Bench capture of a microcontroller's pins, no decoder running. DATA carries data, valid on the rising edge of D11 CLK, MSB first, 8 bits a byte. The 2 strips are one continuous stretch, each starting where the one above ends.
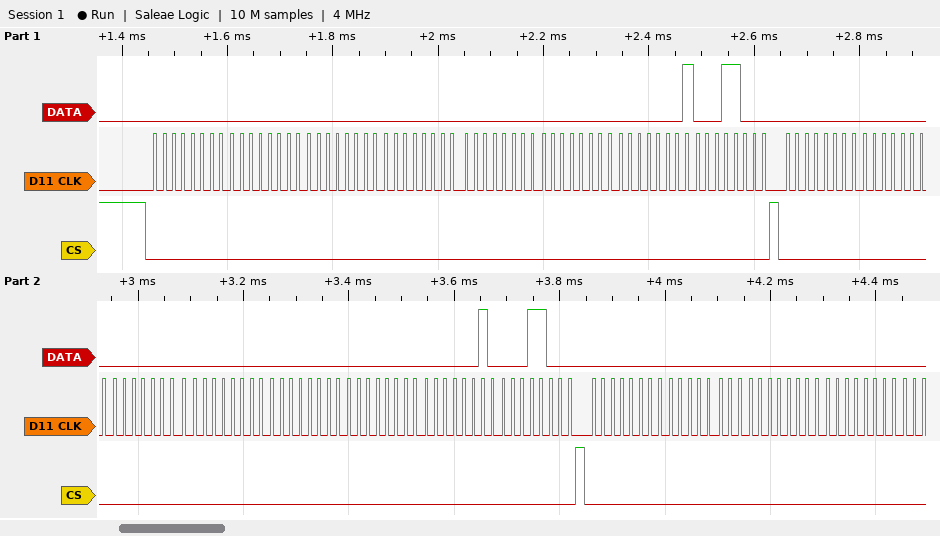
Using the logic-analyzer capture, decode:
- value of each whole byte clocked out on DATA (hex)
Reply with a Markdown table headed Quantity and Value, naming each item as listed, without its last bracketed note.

| Quantity | Value |
|---|---|
| value of each whole byte clocked out on DATA | 00 00 00 00 00 00 01 18 00 00 00 00 00 00 02 18 00 00 00 00 |
